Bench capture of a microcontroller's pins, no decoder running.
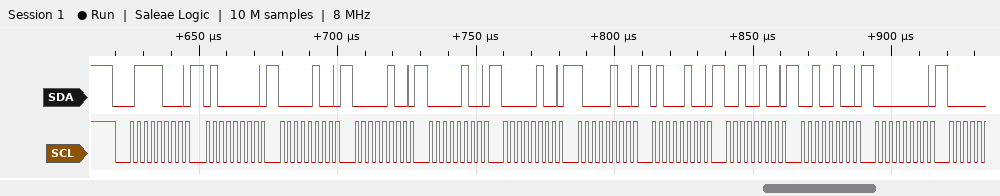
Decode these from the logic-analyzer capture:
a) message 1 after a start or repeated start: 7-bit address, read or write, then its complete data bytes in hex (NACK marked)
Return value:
0x3C write: 40 04 04 04 04 84 44 24 24 00
